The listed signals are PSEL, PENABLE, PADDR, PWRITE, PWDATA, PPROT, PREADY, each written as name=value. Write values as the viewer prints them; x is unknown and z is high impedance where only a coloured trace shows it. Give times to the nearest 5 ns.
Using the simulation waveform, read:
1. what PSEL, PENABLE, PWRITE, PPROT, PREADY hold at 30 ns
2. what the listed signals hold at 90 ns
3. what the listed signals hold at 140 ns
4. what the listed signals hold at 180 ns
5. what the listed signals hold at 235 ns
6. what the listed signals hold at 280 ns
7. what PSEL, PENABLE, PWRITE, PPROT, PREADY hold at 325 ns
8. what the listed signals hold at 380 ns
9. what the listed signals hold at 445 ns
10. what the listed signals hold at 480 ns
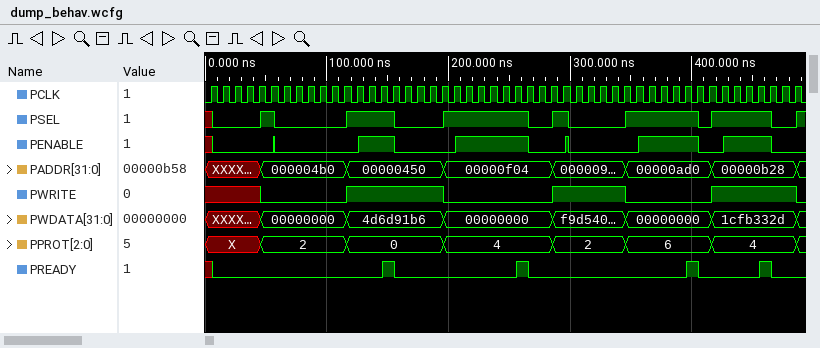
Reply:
PSEL=0, PENABLE=0, PWRITE=x, PPROT=X, PREADY=0
PSEL=0, PENABLE=0, PADDR=000004b0, PWRITE=0, PWDATA=00000000, PPROT=2, PREADY=0
PSEL=1, PENABLE=1, PADDR=00000450, PWRITE=1, PWDATA=4d6d91b6, PPROT=0, PREADY=0
PSEL=0, PENABLE=0, PADDR=00000450, PWRITE=1, PWDATA=4d6d91b6, PPROT=0, PREADY=0
PSEL=1, PENABLE=1, PADDR=00000f04, PWRITE=0, PWDATA=00000000, PPROT=4, PREADY=0
PSEL=0, PENABLE=0, PADDR=00000f04, PWRITE=0, PWDATA=00000000, PPROT=4, PREADY=0
PSEL=0, PENABLE=0, PWRITE=1, PPROT=2, PREADY=0
PSEL=1, PENABLE=1, PADDR=00000ad0, PWRITE=0, PWDATA=00000000, PPROT=6, PREADY=0
PSEL=1, PENABLE=1, PADDR=00000b28, PWRITE=1, PWDATA=1cfb332d, PPROT=4, PREADY=0
PSEL=0, PENABLE=0, PADDR=00000b28, PWRITE=1, PWDATA=1cfb332d, PPROT=4, PREADY=0
